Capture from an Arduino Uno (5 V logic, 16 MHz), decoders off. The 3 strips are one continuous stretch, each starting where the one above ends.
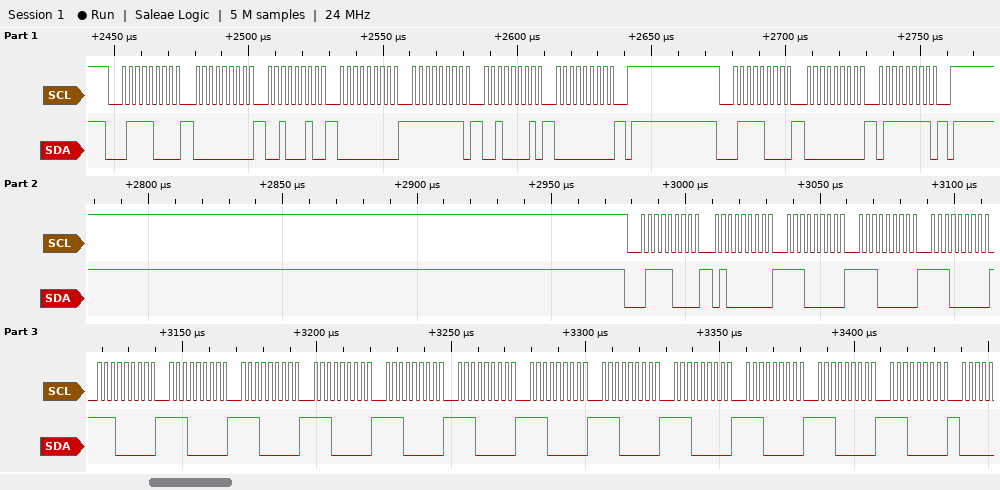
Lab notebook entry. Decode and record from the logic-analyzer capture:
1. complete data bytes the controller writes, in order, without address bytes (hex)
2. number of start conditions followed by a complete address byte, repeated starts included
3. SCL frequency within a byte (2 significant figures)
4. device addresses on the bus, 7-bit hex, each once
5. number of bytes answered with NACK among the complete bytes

00 22 00 FF 21 00 00 7F 40 E0 E0 E0 E0 E0 E0 E0 E0 E0 E0 E0 E0 E0 E0 E0
3
400 kHz
0x3C
0
